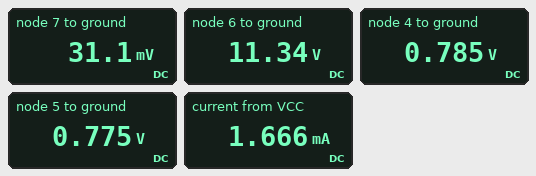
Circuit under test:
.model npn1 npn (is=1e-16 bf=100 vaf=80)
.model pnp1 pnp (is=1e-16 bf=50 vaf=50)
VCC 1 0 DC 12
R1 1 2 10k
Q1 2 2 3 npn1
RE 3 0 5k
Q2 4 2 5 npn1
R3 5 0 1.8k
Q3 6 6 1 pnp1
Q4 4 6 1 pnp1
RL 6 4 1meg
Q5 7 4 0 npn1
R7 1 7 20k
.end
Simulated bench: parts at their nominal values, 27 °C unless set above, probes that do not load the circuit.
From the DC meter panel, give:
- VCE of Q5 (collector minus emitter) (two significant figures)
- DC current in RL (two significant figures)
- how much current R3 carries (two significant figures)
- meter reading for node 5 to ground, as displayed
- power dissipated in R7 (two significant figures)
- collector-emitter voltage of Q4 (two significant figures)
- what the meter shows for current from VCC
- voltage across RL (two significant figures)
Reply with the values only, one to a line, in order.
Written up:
31 mV
11 µA
430 µA
0.775 V
7.2 mW
-11 V
1.666 mA
11 V
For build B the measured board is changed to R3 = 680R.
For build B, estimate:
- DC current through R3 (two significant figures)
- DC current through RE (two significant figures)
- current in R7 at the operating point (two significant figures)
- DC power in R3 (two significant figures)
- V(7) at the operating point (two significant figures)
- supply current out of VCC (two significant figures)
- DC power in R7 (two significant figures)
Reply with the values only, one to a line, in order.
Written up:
940 µA
140 µA
12 µA
600 µW
12 V
1.1 mA
3.0 µW
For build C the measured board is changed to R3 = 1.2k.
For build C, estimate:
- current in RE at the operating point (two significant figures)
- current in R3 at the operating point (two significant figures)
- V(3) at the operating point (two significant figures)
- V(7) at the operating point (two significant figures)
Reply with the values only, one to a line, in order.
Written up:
160 µA
640 µA
820 mV
38 mV
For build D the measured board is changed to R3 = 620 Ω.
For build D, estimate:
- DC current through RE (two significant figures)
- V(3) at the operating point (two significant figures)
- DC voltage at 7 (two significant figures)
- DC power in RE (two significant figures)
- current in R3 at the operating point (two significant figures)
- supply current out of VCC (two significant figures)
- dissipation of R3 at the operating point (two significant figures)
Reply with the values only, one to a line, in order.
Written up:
130 µA
660 mV
12 V
87 µW
950 µA
1.1 mA
560 µW
